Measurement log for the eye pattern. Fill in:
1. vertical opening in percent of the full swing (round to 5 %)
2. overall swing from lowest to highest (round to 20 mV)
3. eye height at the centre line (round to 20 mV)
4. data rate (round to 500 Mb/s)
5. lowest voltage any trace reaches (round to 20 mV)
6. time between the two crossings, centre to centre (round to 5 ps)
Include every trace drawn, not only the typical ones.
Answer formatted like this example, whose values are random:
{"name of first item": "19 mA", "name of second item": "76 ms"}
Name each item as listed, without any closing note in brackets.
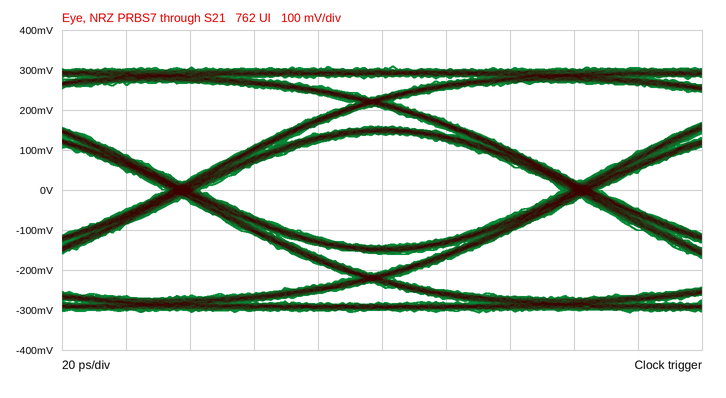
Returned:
{"vertical opening in percent of the full swing": "45 %", "overall swing from lowest to highest": "620 mV", "eye height at the centre line": "280 mV", "data rate": "8.0 Gb/s", "lowest voltage any trace reaches": "-300 mV", "time between the two crossings, centre to centre": "125 ps"}
